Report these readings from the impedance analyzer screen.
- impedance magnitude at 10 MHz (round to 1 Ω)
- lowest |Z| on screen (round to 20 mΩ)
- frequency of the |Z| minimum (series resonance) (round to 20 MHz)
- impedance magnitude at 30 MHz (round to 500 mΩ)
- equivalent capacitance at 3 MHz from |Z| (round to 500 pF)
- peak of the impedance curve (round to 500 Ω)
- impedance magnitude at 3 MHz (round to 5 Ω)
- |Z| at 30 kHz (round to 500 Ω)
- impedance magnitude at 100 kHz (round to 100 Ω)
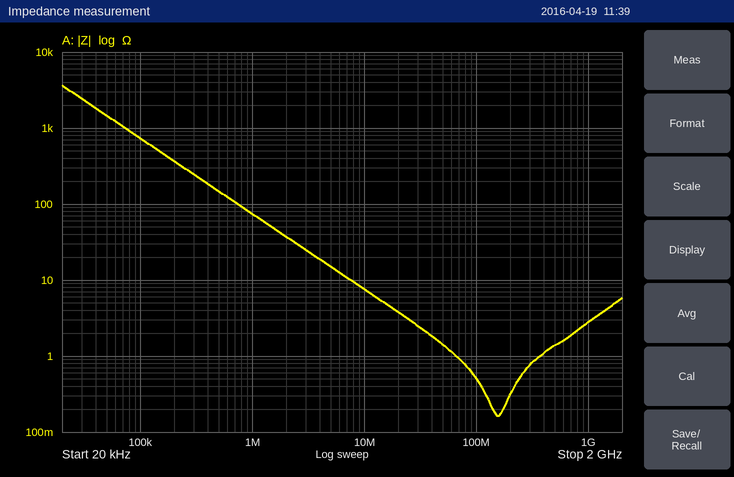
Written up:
8 Ω
160 mΩ
160 MHz
2.5 Ω
2.0 nF
3.5 kΩ
25 Ω
2.5 kΩ
700 Ω
